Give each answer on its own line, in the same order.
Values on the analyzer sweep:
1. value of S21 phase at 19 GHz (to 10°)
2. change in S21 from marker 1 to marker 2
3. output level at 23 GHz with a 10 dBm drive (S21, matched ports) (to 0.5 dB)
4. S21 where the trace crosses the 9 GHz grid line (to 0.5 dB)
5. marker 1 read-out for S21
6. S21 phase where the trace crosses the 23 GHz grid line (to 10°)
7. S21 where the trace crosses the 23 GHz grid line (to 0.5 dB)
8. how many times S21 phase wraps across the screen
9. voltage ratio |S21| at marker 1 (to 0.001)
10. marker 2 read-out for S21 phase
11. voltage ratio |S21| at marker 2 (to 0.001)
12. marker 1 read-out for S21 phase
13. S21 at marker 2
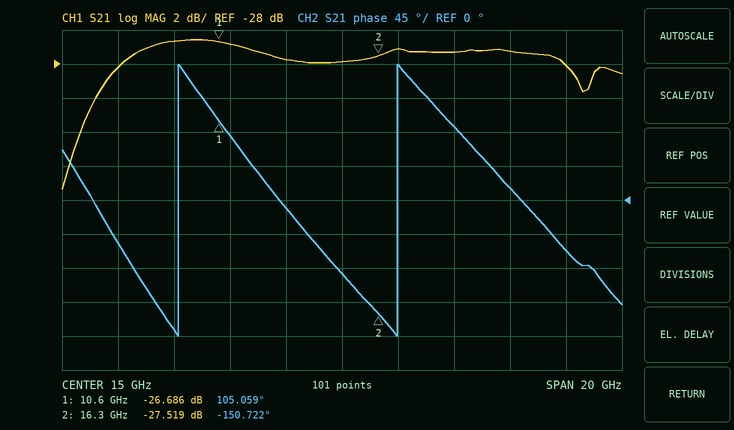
100°
-0.833 dB
-18.0 dBm
-26.5 dB
-26.686 dB
-70°
-28.0 dB
2
0.046
-150.722°
0.042
105.059°
-27.519 dB
